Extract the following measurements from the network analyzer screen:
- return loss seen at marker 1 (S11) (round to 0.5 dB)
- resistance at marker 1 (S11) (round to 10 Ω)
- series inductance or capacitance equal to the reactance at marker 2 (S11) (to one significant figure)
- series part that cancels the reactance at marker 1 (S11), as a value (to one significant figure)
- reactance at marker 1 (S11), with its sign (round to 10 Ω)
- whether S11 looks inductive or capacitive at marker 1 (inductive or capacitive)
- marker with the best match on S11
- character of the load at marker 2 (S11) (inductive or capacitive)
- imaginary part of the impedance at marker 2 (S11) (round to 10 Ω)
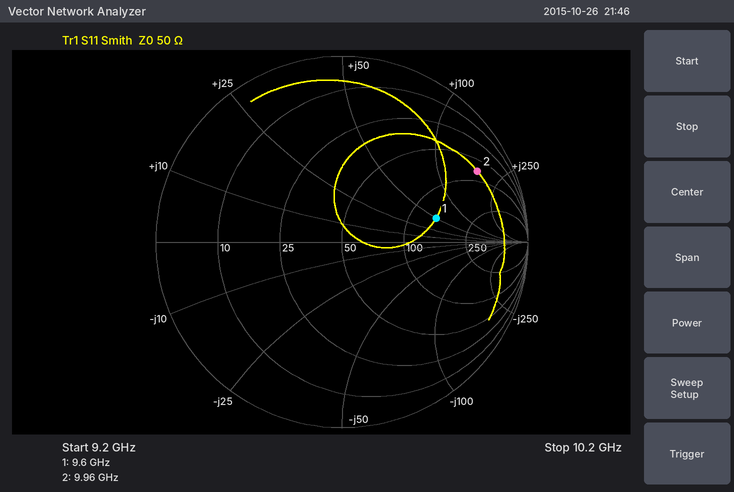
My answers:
5.5 dB
140 Ω
3 nH
300 fF
+50 Ω
inductive
marker 1
inductive
+170 Ω
